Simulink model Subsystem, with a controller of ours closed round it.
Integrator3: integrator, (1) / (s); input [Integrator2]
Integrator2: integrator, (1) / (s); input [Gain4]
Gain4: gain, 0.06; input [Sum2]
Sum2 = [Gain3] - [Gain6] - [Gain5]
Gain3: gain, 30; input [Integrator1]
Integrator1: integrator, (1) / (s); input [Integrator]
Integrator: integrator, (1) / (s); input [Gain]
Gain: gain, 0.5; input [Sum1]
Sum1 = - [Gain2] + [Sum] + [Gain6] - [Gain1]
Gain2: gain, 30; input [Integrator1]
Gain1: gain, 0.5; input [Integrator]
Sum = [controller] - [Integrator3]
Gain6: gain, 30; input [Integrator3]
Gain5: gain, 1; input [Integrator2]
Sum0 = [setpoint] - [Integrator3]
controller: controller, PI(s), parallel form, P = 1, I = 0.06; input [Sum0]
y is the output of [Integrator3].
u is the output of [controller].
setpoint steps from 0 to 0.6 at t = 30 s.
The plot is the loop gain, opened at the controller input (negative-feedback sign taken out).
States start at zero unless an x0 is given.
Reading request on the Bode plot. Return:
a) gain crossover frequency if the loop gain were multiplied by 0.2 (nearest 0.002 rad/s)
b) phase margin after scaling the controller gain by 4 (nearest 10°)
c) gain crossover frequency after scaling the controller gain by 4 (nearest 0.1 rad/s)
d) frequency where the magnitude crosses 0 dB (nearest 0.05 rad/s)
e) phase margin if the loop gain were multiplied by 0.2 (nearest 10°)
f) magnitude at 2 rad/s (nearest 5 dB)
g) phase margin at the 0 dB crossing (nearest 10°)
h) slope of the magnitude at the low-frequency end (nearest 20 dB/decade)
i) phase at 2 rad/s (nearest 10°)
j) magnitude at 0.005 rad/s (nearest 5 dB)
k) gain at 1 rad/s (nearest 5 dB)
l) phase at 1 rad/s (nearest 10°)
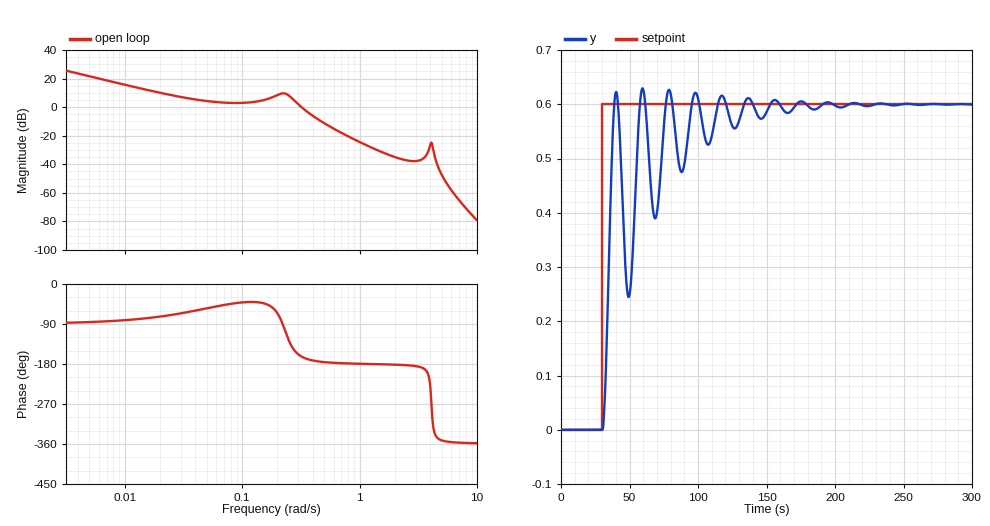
0.012 rad/s
0°
0.5 rad/s
0.30 rad/s
100°
-35 dB
20°
-20 dB/decade
-180°
20 dB
-25 dB
-180°
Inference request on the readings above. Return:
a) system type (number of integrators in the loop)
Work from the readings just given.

1
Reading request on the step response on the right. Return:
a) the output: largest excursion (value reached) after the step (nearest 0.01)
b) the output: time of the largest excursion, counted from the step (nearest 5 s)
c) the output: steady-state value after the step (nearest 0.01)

0.63
30 s
0.60
